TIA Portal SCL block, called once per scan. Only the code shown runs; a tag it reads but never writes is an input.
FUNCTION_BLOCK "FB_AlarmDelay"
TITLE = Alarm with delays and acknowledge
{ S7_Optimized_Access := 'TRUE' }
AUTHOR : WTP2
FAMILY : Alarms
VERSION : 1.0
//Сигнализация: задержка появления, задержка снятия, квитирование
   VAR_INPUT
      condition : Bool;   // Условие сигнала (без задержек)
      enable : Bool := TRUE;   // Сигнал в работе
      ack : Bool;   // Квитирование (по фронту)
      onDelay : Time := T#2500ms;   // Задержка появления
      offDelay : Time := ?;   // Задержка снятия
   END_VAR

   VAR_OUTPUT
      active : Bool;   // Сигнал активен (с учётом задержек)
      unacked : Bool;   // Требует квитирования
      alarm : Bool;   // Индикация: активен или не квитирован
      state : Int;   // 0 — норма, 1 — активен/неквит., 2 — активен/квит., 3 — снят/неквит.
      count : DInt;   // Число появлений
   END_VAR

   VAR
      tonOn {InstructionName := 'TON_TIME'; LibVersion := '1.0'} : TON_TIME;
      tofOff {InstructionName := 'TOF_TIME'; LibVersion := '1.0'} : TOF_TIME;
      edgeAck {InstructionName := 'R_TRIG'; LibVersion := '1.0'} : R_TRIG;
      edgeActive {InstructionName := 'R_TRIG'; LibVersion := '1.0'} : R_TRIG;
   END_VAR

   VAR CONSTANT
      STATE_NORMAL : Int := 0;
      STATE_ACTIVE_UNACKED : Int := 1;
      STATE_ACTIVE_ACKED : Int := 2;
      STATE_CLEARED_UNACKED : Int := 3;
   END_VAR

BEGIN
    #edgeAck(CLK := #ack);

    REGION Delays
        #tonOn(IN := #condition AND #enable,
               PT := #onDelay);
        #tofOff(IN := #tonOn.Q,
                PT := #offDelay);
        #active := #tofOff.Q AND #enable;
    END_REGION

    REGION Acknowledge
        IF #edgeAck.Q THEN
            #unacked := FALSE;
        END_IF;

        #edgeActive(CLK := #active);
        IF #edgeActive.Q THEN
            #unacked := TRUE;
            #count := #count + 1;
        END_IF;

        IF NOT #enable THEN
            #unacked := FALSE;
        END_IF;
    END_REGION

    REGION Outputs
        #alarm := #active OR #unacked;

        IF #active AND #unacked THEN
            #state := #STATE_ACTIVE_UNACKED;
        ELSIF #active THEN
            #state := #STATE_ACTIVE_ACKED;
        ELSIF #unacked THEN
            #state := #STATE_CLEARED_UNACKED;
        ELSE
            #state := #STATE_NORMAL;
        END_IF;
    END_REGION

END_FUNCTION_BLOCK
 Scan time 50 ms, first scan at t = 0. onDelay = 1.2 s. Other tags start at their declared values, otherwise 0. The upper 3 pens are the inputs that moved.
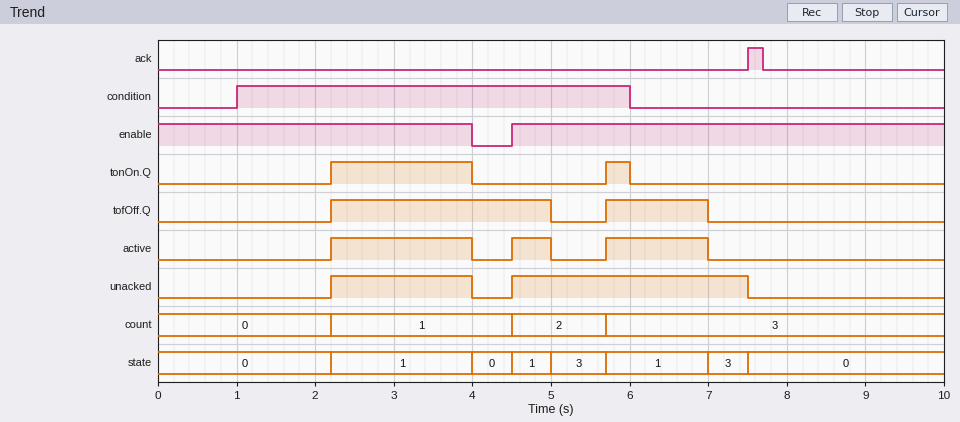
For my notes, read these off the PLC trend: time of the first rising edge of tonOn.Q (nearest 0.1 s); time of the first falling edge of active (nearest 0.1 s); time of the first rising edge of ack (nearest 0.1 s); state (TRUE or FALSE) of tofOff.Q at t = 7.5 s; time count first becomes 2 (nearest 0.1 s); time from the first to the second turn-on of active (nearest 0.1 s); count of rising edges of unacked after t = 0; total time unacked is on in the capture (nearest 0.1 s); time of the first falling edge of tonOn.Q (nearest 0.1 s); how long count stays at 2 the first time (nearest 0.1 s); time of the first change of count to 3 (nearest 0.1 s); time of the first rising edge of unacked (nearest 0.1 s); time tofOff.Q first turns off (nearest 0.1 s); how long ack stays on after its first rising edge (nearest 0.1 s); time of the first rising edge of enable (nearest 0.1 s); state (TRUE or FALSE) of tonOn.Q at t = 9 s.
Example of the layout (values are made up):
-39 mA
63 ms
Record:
2.2 s
4.0 s
7.5 s
FALSE
4.5 s
2.3 s
2
4.8 s
4.0 s
1.2 s
5.7 s
2.2 s
5.0 s
0.2 s
4.5 s
FALSE
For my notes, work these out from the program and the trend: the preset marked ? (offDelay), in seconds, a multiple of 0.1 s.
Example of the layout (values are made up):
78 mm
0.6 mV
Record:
1.0 s
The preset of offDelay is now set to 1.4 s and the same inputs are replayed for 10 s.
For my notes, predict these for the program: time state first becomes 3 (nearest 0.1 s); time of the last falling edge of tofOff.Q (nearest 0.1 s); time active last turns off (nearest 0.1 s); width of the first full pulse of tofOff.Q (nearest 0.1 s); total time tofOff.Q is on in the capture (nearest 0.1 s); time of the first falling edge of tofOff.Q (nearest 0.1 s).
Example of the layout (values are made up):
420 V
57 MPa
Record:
5.4 s
7.4 s
7.4 s
3.2 s
4.9 s
5.4 s
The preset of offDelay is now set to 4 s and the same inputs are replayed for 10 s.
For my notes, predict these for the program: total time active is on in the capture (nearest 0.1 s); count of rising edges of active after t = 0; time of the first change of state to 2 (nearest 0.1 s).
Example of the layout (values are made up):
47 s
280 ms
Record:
7.3 s
2
7.5 s
